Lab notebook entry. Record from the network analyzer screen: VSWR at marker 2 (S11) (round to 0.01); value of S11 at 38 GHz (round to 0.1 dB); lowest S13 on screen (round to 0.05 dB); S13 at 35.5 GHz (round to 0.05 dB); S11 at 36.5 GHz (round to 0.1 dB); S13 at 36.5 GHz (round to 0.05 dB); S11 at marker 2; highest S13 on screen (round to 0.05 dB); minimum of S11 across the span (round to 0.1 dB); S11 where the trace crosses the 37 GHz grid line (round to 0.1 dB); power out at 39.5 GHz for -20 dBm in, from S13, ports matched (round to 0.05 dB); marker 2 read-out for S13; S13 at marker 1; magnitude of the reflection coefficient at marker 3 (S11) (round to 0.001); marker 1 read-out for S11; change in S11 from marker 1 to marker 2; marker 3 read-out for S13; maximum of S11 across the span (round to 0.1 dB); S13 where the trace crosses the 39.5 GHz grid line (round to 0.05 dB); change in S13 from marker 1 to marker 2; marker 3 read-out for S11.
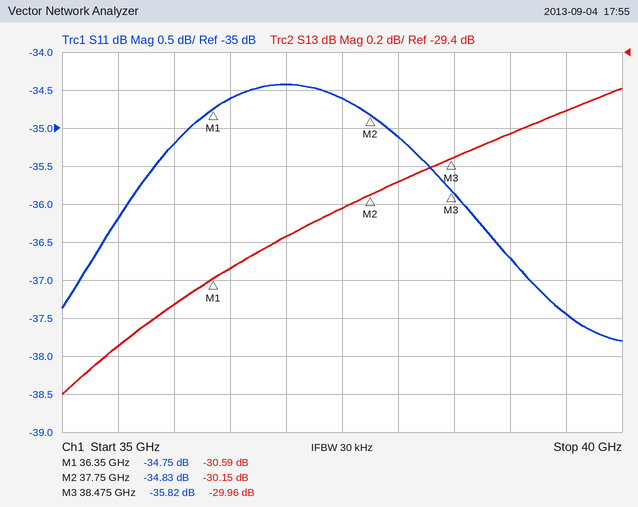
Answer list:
1.04
-35.1 dB
-31.20 dB
-30.95 dB
-34.6 dB
-30.55 dB
-34.83 dB
-29.60 dB
-37.8 dB
-34.4 dB
-49.70 dBm
-30.15 dB
-30.59 dB
0.016
-34.75 dB
-0.08 dB
-29.96 dB
-34.4 dB
-29.70 dB
0.44 dB
-35.82 dB
